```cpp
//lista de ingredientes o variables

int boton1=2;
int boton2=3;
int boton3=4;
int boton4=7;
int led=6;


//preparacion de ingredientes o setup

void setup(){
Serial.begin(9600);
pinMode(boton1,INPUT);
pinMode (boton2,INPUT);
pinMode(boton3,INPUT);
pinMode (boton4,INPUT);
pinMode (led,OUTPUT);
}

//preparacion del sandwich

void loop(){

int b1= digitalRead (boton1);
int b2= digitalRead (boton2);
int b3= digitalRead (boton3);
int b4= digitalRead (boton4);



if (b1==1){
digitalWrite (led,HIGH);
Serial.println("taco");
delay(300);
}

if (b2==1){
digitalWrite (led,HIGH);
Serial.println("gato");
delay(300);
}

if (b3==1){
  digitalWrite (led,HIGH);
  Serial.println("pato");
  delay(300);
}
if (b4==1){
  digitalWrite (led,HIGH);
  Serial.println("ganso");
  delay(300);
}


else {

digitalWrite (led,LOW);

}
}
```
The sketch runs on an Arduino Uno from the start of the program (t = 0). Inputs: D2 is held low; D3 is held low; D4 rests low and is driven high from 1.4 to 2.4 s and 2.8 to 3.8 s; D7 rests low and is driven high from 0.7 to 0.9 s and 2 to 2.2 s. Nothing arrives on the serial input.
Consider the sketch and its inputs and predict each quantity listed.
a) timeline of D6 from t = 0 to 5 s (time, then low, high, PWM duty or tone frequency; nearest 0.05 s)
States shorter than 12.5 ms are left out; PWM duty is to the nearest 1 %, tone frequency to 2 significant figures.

0 s low; 0.7 s high; 1 s low; 1.4 s high; 2.6 s low; 2.8 s high; 4 s low
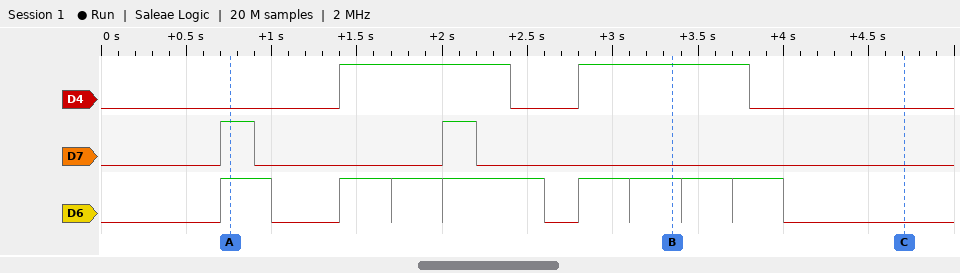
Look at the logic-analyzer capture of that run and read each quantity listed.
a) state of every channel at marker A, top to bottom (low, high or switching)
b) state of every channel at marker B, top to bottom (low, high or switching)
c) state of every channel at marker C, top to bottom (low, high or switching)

D4 low, D7 high, D6 high
D4 high, D7 low, D6 high
D4 low, D7 low, D6 low
